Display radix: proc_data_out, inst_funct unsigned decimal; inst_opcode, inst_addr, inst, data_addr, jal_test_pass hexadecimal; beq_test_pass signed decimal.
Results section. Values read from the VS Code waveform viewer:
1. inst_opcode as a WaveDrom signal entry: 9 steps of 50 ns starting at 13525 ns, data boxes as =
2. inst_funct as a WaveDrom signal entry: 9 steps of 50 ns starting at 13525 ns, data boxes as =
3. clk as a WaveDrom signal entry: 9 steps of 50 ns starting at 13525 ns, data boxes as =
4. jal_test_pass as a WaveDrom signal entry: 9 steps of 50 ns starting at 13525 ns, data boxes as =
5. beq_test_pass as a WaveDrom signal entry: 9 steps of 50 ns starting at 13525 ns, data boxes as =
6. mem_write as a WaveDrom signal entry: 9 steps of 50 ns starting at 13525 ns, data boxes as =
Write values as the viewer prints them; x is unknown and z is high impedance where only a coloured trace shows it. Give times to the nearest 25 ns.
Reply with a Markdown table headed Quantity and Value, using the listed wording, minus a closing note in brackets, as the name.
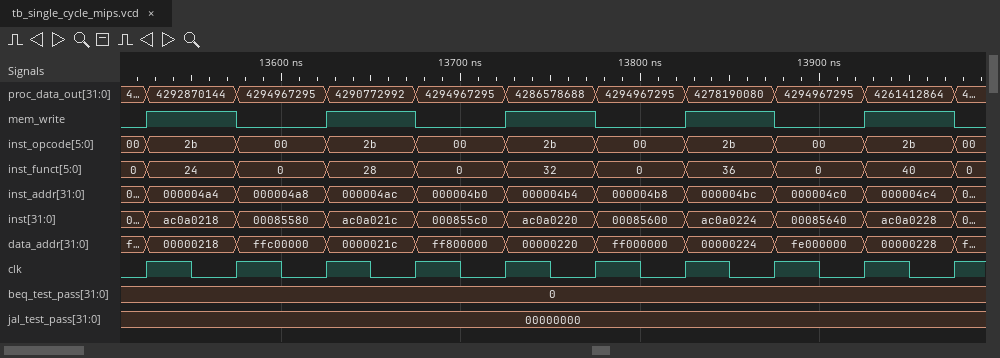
| Quantity | Value |
|---|---|
| inst_opcode as a WaveDrom signal entry: 9 steps of 50 ns starting at 13525 ns, data boxes as = | {name: 'inst_opcode', wave: '=========', data: '2b 00 2b 00 2b 00 2b 00 2b'} |
| inst_funct as a WaveDrom signal entry: 9 steps of 50 ns starting at 13525 ns, data boxes as = | {name: 'inst_funct', wave: '=========', data: '24 0 28 0 32 0 36 0 40'} |
| clk as a WaveDrom signal entry: 9 steps of 50 ns starting at 13525 ns, data boxes as = | {name: 'clk', wave: 'p........'} |
| jal_test_pass as a WaveDrom signal entry: 9 steps of 50 ns starting at 13525 ns, data boxes as = | {name: 'jal_test_pass', wave: '=........', data: '00000000'} |
| beq_test_pass as a WaveDrom signal entry: 9 steps of 50 ns starting at 13525 ns, data boxes as = | {name: 'beq_test_pass', wave: '=........', data: '0'} |
| mem_write as a WaveDrom signal entry: 9 steps of 50 ns starting at 13525 ns, data boxes as = | {name: 'mem_write', wave: '101010101'} |
